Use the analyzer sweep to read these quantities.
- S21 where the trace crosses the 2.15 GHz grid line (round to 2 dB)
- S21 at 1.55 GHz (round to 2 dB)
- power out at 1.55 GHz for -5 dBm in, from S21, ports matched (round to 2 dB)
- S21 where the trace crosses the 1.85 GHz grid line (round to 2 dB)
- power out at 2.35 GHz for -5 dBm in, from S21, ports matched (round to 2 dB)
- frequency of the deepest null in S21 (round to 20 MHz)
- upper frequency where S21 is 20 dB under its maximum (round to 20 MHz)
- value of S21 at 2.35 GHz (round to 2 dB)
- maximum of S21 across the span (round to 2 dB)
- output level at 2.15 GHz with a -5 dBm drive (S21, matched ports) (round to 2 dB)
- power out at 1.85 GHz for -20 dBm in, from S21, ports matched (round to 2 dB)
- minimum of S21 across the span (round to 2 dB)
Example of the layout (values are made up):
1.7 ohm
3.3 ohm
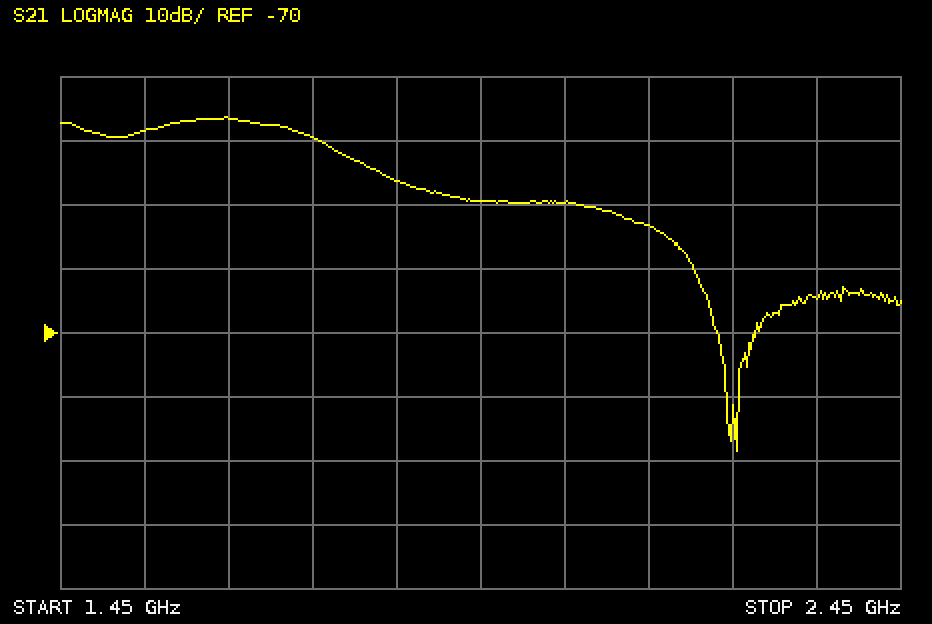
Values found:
-54 dB
-38 dB
-44 dBm
-46 dB
-70 dBm
2.26 GHz
2.18 GHz
-64 dB
-36 dB
-58 dBm
-66 dBm
-88 dB
